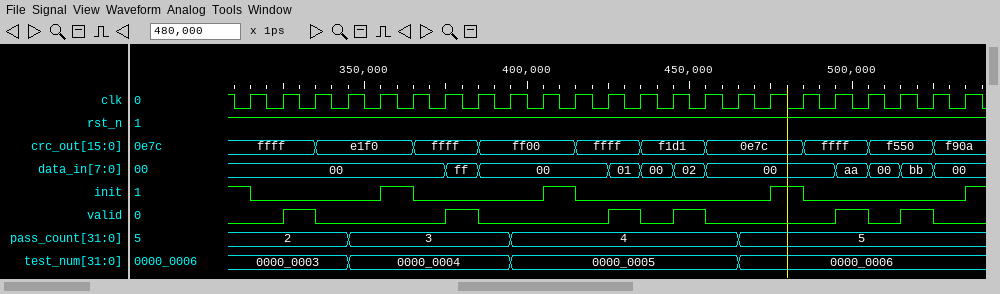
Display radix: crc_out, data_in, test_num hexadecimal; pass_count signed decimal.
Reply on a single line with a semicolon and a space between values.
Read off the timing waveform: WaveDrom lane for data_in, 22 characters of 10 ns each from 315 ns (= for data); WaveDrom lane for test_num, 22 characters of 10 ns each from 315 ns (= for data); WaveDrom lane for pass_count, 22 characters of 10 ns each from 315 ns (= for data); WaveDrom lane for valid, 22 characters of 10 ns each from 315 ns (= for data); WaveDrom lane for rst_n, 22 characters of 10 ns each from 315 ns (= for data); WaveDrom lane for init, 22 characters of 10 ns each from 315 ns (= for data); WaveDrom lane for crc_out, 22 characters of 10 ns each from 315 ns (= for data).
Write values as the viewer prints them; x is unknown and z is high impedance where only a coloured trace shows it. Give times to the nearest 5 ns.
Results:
{name: 'data_in', wave: '=.....==...====...====', data: '00 ff 00 01 00 02 00 aa 00 bb 00'}; {name: 'test_num', wave: '=..=....=......=......', data: '0000_0003 0000_0004 0000_0005 0000_0006'}; {name: 'pass_count', wave: '=..=....=......=......', data: '2 3 4 5'}; {name: 'valid', wave: '010...10...1010...1010'}; {name: 'rst_n', wave: '1.....................'}; {name: 'init', wave: '0...10...10.....10....'}; {name: 'crc_out', wave: '=.=..=.=..=.=.=..=.=.=', data: 'ffff e1f0 ffff ff00 ffff f1d1 0e7c ffff f550 f90a'}
